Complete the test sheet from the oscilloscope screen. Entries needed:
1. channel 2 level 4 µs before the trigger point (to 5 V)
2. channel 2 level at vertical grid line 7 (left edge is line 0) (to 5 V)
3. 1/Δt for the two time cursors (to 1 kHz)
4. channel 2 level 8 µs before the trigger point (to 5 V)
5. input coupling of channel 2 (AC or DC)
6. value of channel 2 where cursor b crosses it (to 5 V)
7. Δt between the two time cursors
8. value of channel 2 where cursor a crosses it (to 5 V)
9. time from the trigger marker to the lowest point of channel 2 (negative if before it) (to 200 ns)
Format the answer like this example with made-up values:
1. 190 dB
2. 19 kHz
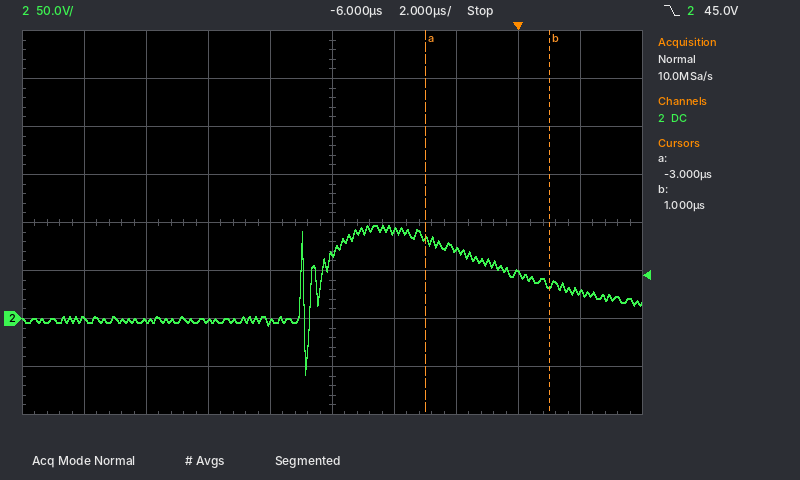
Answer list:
1. 90 V
2. 70 V
3. 250 kHz
4. -5 V
5. DC
6. 35 V
7. 4.0 µs
8. 80 V
9. -6.8 µs
